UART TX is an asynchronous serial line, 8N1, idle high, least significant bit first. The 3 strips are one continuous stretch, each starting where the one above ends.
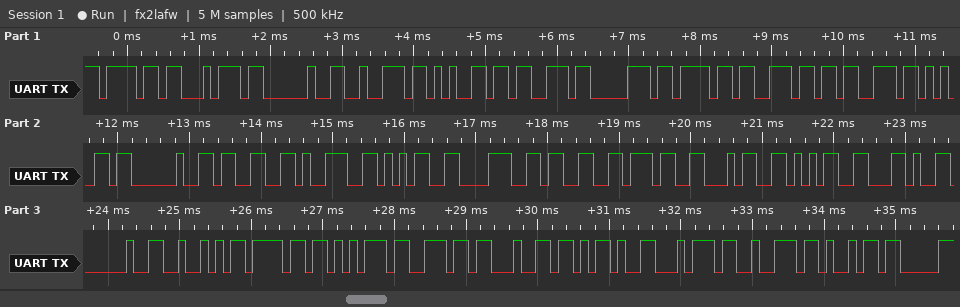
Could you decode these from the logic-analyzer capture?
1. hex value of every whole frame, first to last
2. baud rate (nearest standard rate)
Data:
6F 74 20 72 65 73 70 6F 6E 73 65 20 33 39 35 38 33 37 34 35 2C 20 52 6F 75 6E 64 2D 74 72 69
9600 baud
